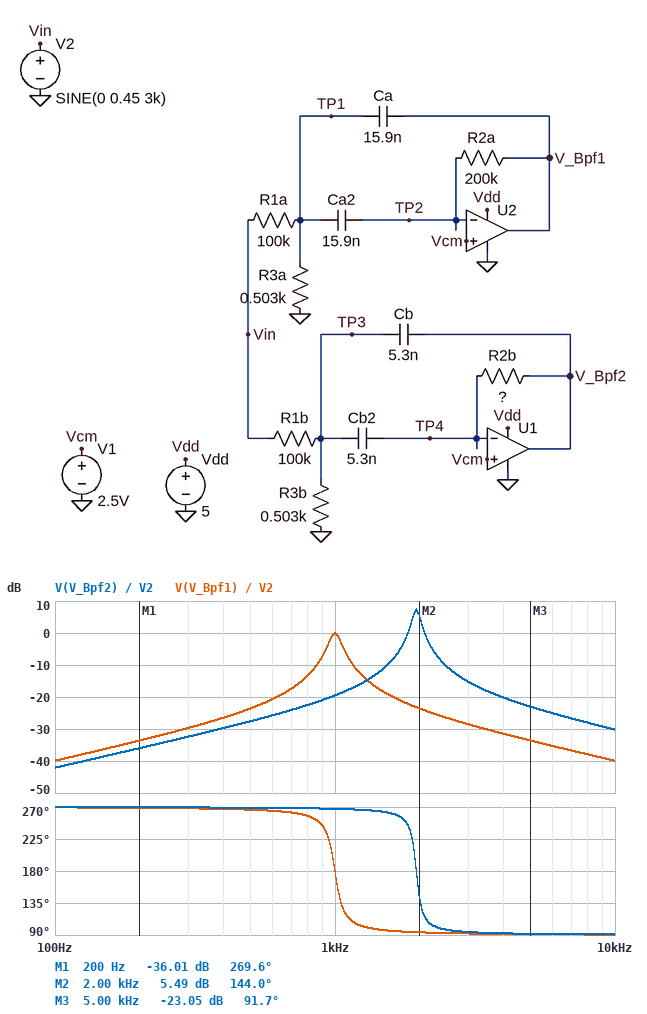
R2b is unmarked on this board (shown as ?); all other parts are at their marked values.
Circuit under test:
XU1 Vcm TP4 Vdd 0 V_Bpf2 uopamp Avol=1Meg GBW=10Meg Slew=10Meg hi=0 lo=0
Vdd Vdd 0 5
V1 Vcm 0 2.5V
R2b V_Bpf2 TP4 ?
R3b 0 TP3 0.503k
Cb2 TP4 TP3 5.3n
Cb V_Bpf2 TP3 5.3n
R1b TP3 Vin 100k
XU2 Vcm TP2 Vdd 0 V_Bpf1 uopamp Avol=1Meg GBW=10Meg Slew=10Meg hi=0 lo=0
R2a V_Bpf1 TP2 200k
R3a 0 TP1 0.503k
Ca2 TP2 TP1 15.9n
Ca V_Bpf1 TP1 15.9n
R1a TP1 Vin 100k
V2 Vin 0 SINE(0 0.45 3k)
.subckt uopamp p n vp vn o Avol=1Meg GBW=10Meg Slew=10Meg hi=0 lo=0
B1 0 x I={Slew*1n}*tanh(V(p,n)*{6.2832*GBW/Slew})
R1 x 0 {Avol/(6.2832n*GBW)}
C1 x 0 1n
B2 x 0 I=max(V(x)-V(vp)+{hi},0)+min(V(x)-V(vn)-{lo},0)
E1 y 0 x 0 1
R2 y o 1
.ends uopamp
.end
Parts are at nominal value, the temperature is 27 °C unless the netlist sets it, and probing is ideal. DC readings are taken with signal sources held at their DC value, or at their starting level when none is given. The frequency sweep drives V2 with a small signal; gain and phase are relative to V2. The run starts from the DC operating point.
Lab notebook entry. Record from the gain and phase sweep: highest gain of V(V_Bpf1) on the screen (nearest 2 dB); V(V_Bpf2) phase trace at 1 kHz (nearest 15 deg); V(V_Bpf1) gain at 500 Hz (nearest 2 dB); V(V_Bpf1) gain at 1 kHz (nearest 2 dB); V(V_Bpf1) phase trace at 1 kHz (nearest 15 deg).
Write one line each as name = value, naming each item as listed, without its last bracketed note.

highest gain of V(V_Bpf1) on the screen = 0 dB
V(V_Bpf2) phase trace at 1 kHz = 270 deg
V(V_Bpf1) gain at 500 Hz = -24 dB
V(V_Bpf1) gain at 1 kHz = 0 dB
V(V_Bpf1) phase trace at 1 kHz = 180 deg
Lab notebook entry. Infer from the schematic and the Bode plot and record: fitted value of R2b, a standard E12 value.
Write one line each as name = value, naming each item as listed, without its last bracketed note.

fitted value of R2b, a standard E12 value = 470 kΩ
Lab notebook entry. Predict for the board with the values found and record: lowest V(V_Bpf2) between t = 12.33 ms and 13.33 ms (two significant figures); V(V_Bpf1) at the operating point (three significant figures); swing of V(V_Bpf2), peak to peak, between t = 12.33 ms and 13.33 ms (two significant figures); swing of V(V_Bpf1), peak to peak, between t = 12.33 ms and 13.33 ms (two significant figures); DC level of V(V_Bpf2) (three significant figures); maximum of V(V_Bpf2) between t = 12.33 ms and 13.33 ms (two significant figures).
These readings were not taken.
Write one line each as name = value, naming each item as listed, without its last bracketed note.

lowest V(V_Bpf2) between t = 12.33 ms and 13.33 ms = 2.4 V
V(V_Bpf1) at the operating point = 2.50 V
swing of V(V_Bpf2), peak to peak, between t = 12.33 ms and 13.33 ms = 160 mV
swing of V(V_Bpf1), peak to peak, between t = 12.33 ms and 13.33 ms = 34 mV
DC level of V(V_Bpf2) = 2.50 V
maximum of V(V_Bpf2) between t = 12.33 ms and 13.33 ms = 2.6 V
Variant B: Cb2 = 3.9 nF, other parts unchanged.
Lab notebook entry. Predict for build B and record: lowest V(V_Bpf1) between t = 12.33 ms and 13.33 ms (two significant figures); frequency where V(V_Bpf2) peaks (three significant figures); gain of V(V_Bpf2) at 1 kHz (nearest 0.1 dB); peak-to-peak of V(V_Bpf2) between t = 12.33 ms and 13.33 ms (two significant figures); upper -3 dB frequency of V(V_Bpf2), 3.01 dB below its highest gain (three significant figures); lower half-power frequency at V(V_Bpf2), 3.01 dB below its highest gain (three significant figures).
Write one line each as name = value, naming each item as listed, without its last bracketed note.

lowest V(V_Bpf1) between t = 12.33 ms and 13.33 ms = 2.5 V
frequency where V(V_Bpf2) peaks = 2.28 kHz
gain of V(V_Bpf2) at 1 kHz = -22.9 dB
peak-to-peak of V(V_Bpf2) between t = 12.33 ms and 13.33 ms = 210 mV
upper -3 dB frequency of V(V_Bpf2), 3.01 dB below its highest gain = 2.35 kHz
lower half-power frequency at V(V_Bpf2), 3.01 dB below its highest gain = 2.20 kHz
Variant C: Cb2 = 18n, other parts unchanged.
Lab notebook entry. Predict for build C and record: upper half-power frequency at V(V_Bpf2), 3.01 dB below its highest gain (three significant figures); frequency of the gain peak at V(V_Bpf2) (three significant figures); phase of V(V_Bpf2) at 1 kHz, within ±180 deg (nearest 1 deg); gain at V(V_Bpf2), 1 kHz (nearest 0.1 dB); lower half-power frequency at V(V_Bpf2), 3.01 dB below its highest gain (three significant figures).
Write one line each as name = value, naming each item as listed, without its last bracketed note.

upper half-power frequency at V(V_Bpf2), 3.01 dB below its highest gain = 1.10 kHz
frequency of the gain peak at V(V_Bpf2) = 1.06 kHz
phase of V(V_Bpf2) at 1 kHz, within ±180 deg = -124 deg
gain at V(V_Bpf2), 1 kHz = 6.1 dB
lower half-power frequency at V(V_Bpf2), 3.01 dB below its highest gain = 1.02 kHz
